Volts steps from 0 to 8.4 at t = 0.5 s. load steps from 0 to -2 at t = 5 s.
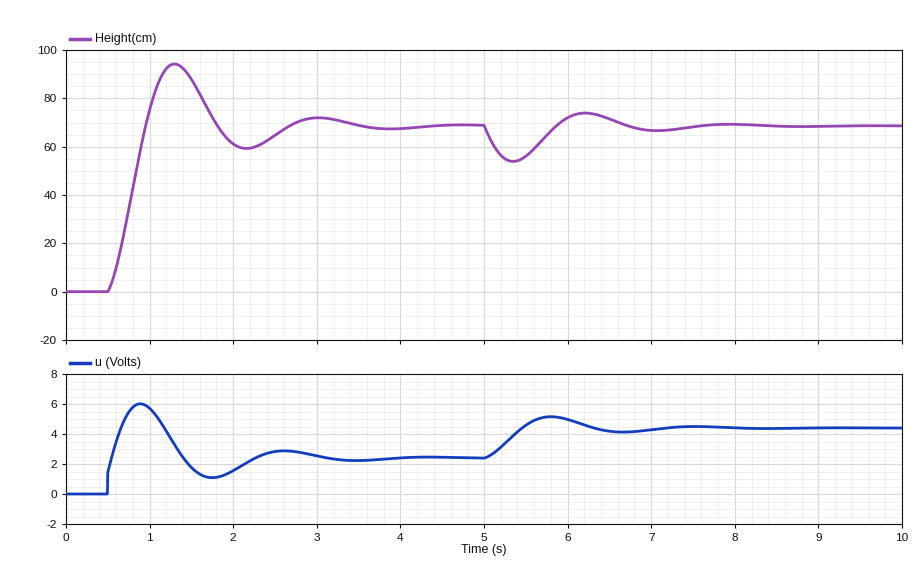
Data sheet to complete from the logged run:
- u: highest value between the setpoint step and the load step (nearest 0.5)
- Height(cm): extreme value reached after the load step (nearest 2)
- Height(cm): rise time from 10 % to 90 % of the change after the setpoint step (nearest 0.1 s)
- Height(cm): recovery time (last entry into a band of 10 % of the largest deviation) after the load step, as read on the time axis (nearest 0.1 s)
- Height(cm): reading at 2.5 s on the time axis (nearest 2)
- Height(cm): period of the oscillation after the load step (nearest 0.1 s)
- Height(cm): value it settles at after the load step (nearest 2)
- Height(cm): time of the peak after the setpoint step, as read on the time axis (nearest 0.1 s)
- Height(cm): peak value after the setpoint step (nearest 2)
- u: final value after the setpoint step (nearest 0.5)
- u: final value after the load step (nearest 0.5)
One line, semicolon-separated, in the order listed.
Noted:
6.0; 54; 0.3 s; 7.3 s; 64; 1.7 s; 68; 1.3 s; 94; 2.5; 4.5
